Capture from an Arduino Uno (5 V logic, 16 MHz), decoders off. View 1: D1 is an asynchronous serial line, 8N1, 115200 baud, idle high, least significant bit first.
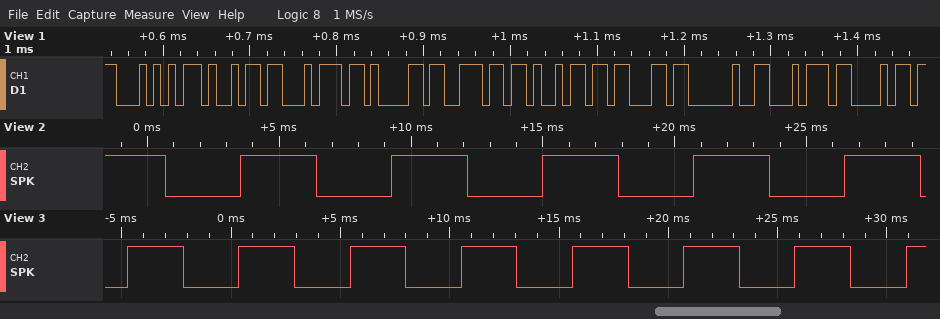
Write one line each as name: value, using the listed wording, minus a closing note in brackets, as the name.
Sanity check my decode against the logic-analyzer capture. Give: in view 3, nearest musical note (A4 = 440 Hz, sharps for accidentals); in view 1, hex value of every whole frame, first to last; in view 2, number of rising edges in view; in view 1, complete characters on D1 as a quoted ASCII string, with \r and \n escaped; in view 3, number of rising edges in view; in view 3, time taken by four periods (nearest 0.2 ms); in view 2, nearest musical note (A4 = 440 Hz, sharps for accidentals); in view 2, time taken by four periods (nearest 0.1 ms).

in view 3, nearest musical note: G3
in view 1, hex value of every whole frame, first to last: 54 69 74 61 6E 69 63 20 74 68
in view 2, number of rising edges in view: 5
in view 1, complete characters on D1 as a quoted ASCII string, with \r and \n escaped: "Titanic th"
in view 3, number of rising edges in view: 8
in view 3, time taken by four periods: 20.4 ms
in view 2, nearest musical note: F3
in view 2, time taken by four periods: 22.9 ms
